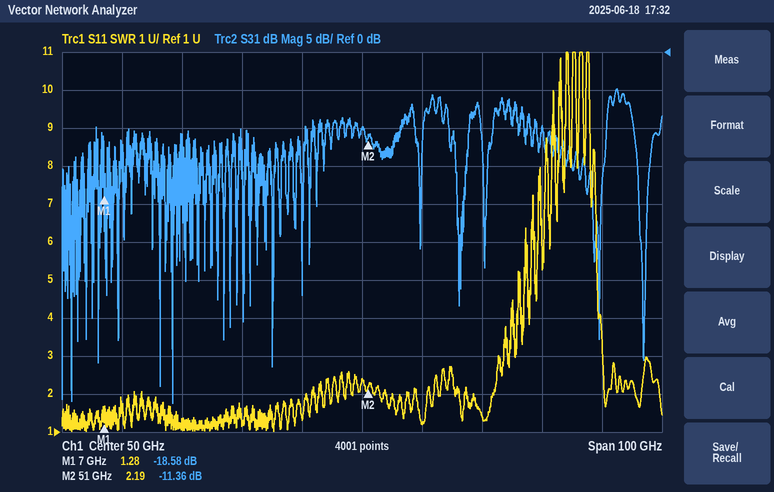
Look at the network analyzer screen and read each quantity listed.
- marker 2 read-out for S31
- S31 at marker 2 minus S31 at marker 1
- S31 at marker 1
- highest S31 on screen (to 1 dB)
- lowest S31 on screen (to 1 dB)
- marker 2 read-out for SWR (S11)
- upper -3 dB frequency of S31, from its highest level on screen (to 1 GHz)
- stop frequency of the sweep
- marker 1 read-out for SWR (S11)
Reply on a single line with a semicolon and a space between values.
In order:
-11.36 dB; 7.22 dB; -18.58 dB; -5 dB; -46 dB; 2.19; 95 GHz; 100 GHz; 1.28
